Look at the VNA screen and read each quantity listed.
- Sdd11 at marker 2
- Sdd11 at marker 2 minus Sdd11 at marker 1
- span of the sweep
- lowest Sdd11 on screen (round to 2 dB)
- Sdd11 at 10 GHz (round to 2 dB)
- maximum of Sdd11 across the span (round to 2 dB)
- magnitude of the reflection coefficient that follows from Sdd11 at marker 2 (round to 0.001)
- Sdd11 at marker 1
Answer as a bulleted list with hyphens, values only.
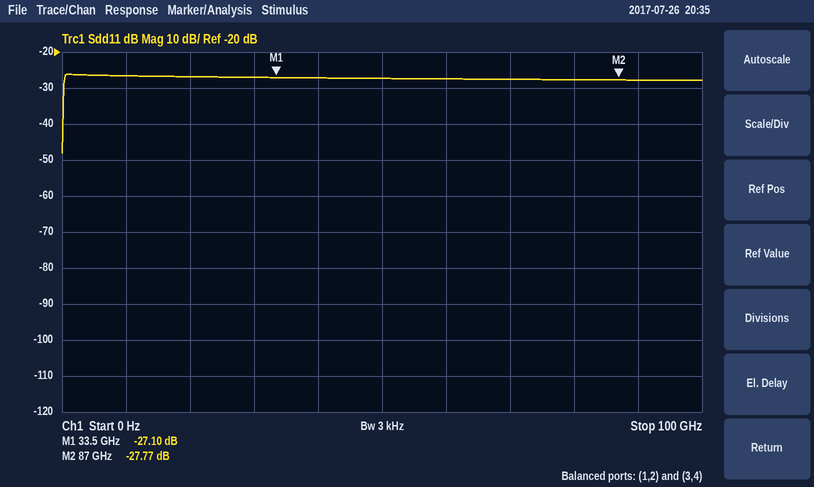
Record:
- -27.77 dB
- -0.67 dB
- 100 GHz
- -48 dB
- -26 dB
- -26 dB
- 0.041
- -27.10 dB
